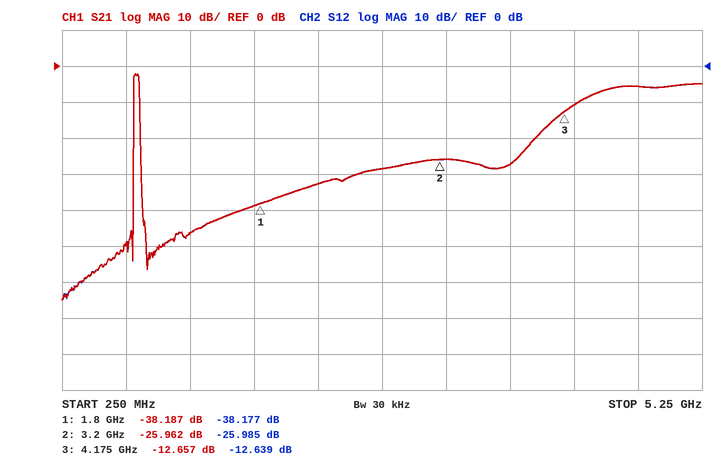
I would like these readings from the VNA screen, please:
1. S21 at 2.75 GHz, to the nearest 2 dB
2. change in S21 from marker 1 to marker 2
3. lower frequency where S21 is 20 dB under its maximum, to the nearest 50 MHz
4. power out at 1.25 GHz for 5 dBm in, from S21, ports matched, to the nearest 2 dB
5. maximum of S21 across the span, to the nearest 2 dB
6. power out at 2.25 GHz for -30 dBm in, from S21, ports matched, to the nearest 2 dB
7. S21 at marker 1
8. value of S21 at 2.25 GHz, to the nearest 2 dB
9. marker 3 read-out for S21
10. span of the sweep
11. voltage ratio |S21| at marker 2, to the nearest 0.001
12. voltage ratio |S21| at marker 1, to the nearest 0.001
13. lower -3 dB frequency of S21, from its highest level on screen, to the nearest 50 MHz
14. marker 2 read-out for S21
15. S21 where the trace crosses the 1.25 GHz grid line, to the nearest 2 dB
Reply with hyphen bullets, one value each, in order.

- -28 dB
- 12.225 dB
- 800 MHz
- -42 dBm
- -2 dB
- -62 dBm
- -38.187 dB
- -32 dB
- -12.657 dB
- 5 GHz
- 0.050
- 0.012
- 800 MHz
- -25.962 dB
- -46 dB
